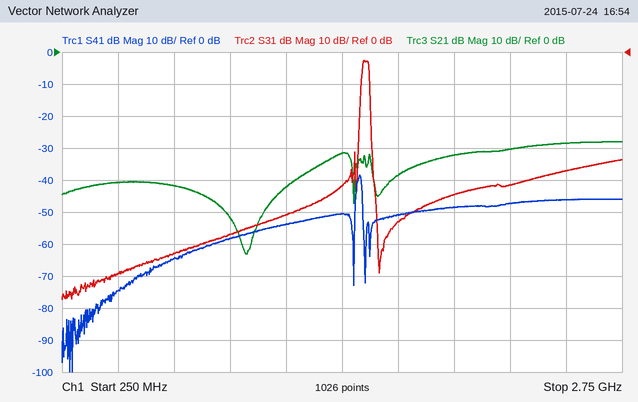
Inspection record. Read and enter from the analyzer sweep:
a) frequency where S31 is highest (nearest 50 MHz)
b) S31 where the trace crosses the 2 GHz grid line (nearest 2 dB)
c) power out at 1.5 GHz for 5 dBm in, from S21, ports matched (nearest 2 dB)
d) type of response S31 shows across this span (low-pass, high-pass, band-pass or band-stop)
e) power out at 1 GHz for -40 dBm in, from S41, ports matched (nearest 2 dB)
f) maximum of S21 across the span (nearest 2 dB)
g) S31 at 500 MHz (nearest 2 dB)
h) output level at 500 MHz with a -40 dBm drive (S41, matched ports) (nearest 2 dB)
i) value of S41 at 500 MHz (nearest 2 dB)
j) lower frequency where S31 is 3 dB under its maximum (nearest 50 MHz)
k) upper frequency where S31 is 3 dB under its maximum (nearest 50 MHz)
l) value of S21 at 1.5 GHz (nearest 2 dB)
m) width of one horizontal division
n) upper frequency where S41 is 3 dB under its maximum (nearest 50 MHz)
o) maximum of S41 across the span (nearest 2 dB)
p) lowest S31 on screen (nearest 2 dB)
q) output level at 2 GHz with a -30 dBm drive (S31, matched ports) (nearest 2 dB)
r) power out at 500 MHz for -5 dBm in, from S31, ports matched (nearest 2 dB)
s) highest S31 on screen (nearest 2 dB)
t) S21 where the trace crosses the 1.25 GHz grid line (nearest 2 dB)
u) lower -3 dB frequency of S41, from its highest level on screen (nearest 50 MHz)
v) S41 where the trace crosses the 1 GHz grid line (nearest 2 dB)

1.60 GHz
-44 dB
-26 dBm
band-pass
-98 dBm
-28 dB
-70 dB
-114 dBm
-74 dB
1.60 GHz
1.60 GHz
-32 dB
250 MHz
1.60 GHz
-38 dB
-78 dB
-74 dBm
-74 dBm
-2 dB
-42 dB
1.55 GHz
-58 dB
